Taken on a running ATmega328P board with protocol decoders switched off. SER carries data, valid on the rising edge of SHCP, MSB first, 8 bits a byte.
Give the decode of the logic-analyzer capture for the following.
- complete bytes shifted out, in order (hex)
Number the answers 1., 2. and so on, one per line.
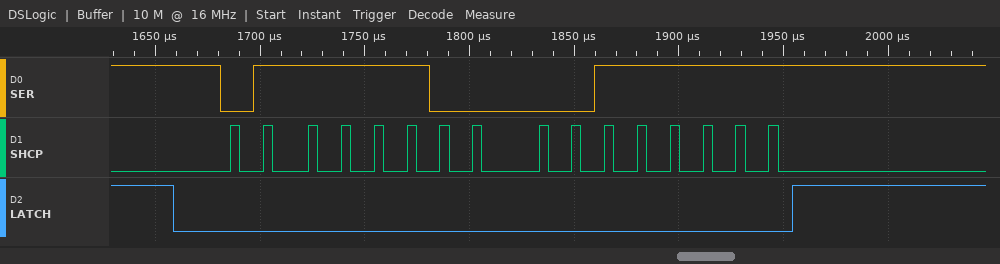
1. 0x7C 0x3F
